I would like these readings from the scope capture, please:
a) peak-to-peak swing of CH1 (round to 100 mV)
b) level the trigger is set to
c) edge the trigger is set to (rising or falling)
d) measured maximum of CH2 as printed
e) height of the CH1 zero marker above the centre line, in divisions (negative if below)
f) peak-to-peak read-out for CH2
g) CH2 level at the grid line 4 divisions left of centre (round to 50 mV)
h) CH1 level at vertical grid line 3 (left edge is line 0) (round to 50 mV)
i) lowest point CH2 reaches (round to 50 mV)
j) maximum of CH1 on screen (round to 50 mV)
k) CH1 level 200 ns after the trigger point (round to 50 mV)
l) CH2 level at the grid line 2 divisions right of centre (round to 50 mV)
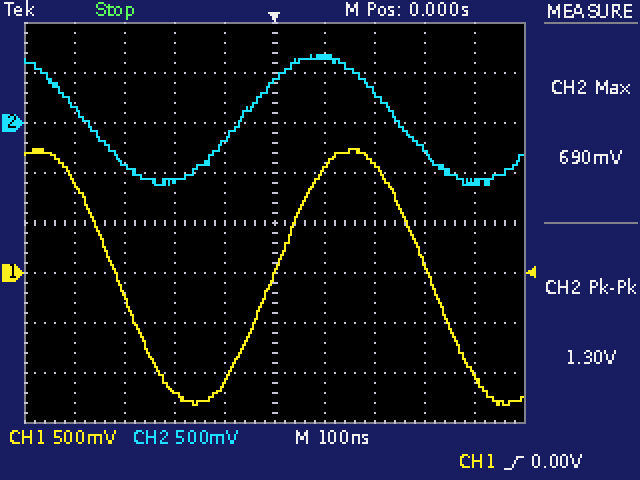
2.60 V
0.00 V
rising
690 mV
-1.0 div
1.30 V
150 mV
-1.20 V
-600 mV
1.25 V
1.10 V
300 mV
